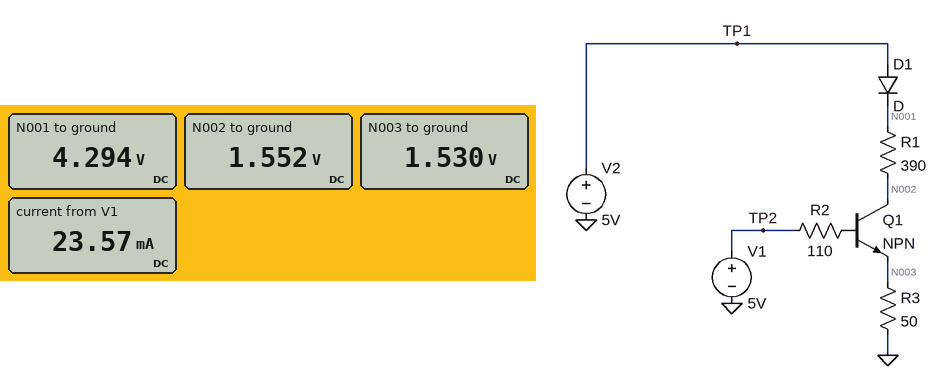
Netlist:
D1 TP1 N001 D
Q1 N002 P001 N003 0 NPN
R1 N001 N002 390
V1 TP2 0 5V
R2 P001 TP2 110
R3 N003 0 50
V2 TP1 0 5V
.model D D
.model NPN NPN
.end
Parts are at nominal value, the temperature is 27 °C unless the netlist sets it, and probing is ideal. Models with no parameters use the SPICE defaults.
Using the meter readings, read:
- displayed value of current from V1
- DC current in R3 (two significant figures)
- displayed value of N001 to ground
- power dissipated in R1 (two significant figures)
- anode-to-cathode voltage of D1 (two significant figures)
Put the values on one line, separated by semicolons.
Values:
23.57 mA; 31 mA; 4.294 V; 19 mW; 710 mV
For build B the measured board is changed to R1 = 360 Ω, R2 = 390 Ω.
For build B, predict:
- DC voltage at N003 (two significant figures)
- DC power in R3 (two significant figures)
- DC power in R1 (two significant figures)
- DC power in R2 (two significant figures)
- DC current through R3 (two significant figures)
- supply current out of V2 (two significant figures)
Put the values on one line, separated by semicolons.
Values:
890 mV; 16 mW; 32 mW; 27 mW; 18 mA; 9.4 mA
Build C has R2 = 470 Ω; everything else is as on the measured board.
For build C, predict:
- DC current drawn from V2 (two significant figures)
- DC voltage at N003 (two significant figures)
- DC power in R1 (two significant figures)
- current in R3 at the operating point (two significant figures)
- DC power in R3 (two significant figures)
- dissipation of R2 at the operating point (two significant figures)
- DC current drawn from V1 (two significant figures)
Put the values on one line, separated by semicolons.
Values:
8.9 mA; 800 mV; 31 mW; 16 mA; 13 mW; 24 mW; 7.1 mA
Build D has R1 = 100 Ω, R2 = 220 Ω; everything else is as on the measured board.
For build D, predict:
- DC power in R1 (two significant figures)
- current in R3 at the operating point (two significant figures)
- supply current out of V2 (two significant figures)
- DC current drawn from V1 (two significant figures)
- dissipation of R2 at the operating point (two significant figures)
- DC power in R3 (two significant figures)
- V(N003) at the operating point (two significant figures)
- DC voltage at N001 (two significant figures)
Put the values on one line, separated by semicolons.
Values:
60 mW; 35 mA; 25 mA; 11 mA; 25 mW; 62 mW; 1.8 V; 4.3 V
